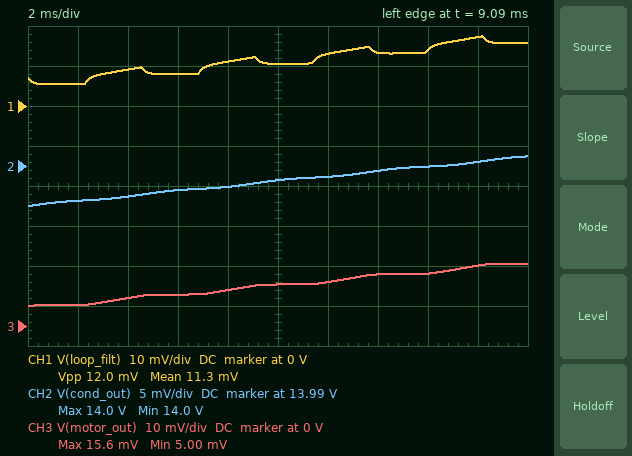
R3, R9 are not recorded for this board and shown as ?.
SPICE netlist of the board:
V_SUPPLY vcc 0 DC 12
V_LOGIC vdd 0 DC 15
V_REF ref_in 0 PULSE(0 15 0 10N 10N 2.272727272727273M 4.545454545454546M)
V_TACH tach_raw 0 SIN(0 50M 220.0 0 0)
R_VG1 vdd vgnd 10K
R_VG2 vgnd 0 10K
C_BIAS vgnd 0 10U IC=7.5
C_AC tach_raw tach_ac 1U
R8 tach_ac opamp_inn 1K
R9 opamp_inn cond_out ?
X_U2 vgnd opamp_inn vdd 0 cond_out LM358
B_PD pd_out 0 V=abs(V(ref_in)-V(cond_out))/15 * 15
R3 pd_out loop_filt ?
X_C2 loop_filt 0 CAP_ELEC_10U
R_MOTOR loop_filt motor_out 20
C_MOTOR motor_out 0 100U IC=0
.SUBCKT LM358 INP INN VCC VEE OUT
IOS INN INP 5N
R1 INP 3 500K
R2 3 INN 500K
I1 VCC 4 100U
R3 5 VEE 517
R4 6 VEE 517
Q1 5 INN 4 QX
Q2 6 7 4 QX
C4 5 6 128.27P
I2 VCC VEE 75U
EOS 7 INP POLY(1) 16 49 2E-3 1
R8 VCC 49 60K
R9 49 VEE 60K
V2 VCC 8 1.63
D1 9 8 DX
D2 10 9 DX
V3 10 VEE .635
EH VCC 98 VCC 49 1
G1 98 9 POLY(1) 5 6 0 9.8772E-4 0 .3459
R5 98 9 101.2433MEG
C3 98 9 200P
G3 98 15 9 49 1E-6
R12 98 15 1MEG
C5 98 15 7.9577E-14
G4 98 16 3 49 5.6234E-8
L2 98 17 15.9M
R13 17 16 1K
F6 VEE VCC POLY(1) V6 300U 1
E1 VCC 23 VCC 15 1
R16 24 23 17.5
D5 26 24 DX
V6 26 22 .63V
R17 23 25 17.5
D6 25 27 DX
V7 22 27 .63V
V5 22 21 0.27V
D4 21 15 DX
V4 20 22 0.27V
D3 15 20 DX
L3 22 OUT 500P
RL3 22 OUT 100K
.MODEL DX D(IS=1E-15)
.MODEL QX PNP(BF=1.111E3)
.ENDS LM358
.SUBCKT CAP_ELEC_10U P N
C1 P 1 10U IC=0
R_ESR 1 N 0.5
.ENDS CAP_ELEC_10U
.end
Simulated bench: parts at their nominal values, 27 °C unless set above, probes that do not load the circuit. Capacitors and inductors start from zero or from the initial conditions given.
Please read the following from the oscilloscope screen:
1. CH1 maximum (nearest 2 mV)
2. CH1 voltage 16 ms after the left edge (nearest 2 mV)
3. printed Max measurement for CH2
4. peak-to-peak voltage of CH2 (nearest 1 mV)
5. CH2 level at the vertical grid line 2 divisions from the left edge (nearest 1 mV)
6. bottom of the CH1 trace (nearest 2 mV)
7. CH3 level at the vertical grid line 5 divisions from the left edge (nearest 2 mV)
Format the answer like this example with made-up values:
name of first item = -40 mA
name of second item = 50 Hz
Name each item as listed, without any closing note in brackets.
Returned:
CH1 maximum = 18 mV
CH1 voltage 16 ms after the left edge = 14 mV
printed Max measurement for CH2 = 14.0 V
peak-to-peak voltage of CH2 = 6 mV
CH2 level at the vertical grid line 2 divisions from the left edge = 13.986 V
bottom of the CH1 trace = 6 mV
CH3 level at the vertical grid line 5 divisions from the left edge = 10 mV
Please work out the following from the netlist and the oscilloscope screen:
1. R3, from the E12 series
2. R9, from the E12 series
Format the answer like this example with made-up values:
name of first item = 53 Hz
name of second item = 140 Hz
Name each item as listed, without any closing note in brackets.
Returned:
R3, from the E12 series = 120 kΩ
R9, from the E12 series = 82 kΩ
